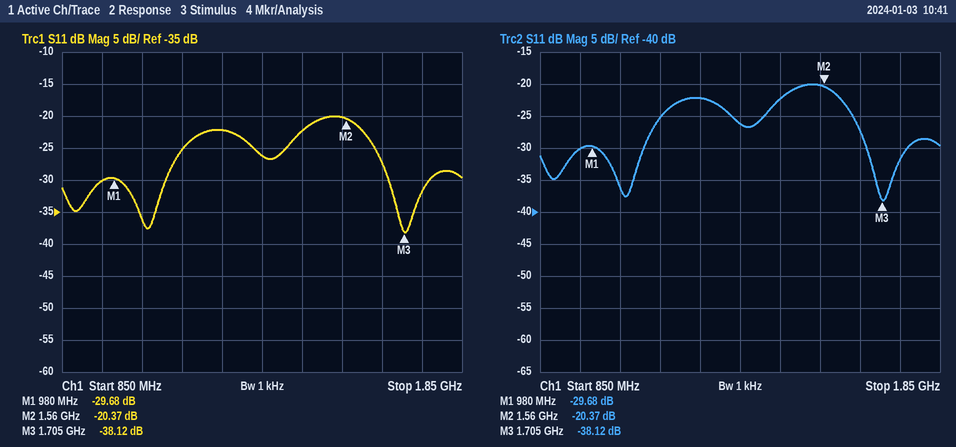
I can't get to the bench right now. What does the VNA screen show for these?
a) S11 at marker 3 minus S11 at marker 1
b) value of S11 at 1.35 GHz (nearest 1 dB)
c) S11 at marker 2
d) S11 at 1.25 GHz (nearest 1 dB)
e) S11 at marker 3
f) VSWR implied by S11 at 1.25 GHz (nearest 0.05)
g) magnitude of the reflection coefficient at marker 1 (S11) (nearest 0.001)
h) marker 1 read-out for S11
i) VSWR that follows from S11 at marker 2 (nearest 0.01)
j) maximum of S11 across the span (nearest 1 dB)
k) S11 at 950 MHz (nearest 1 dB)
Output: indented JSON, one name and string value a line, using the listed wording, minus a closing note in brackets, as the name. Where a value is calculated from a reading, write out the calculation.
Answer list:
{
  "S11 at marker 3 minus S11 at marker 1": "-38.12 − (-29.68) = -8.44 dB",
  "value of S11 at 1.35 GHz": "-26 dB",
  "S11 at marker 2": "-20.37 dB",
  "S11 at 1.25 GHz": "-22 dB",
  "S11 at marker 3": "-38.12 dB",
  "VSWR implied by S11 at 1.25 GHz": "|Γ| = 10^(-22/20) = 0.0794; VSWR = (1 + 0.0794)/(1 − 0.0794) ≈ 1.17, so 1.15 to the nearest 0.05",
  "magnitude of the reflection coefficient at marker 1 (S11)": "10^(-29.68/20) ≈ 0.033",
  "marker 1 read-out for S11": "-29.68 dB",
  "VSWR that follows from S11 at marker 2": "(1 + 0.0958)/(1 − 0.0958) ≈ 1.21",
  "maximum of S11 across the span": "-20 dB",
  "S11 at 950 MHz": "-30 dB"
}
